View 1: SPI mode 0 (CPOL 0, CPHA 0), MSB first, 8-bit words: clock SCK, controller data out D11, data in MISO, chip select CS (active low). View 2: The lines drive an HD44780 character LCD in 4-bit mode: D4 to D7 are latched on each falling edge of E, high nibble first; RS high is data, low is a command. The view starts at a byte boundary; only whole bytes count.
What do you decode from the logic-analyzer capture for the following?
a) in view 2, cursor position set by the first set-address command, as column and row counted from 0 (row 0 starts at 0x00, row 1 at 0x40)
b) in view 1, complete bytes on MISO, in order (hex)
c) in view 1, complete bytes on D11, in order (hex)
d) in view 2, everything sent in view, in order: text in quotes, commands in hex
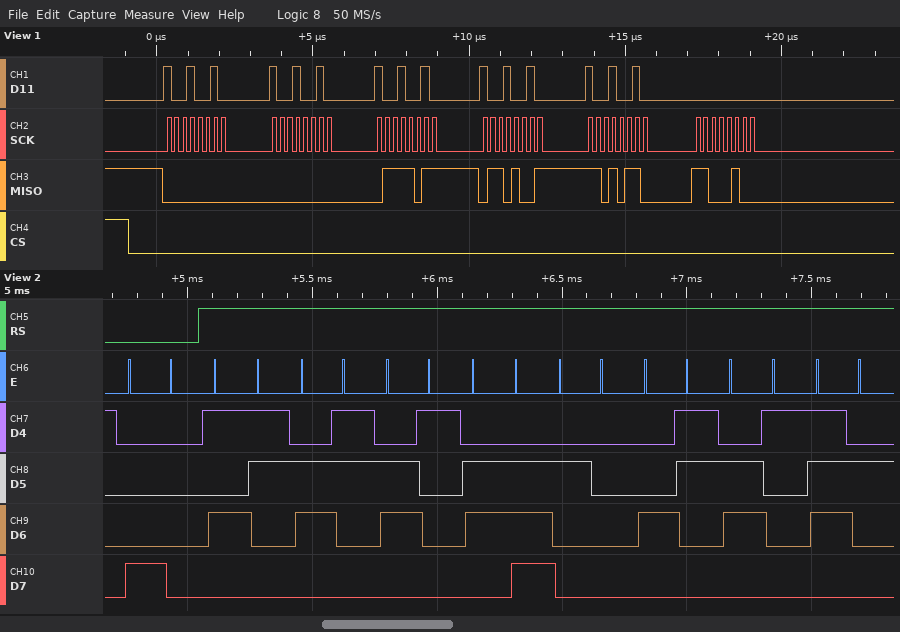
column 0, row 0
00 00 7B 69 D6 C4
92 92 92 92 92 00
0x80 "Scan Car"
